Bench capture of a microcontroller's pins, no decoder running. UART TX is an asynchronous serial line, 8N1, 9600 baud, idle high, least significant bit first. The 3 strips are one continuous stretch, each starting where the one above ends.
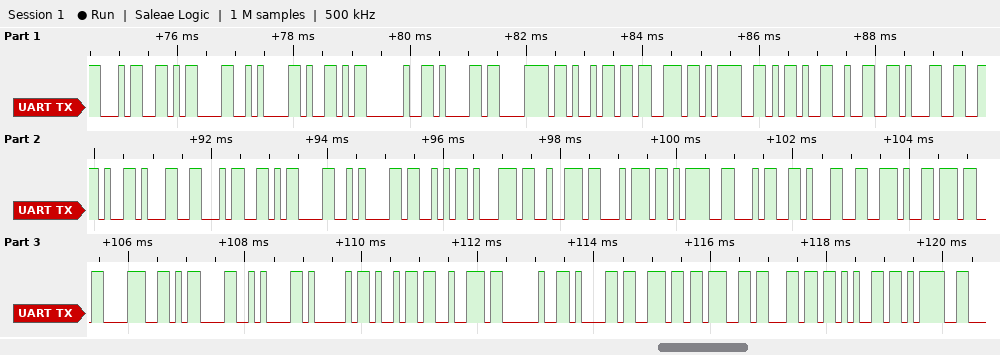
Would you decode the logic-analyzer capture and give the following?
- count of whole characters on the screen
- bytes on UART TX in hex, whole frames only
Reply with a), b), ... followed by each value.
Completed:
a) 40
b) 34 0D 0A 59 20 61 78 69 73 3D 2D 32 31 2E 31 34 0D 0A 53 71 72 74 3D 34 31 2E 37 38 0D 0A 41 69 72 20 61 6E 67 6C 65 3D
